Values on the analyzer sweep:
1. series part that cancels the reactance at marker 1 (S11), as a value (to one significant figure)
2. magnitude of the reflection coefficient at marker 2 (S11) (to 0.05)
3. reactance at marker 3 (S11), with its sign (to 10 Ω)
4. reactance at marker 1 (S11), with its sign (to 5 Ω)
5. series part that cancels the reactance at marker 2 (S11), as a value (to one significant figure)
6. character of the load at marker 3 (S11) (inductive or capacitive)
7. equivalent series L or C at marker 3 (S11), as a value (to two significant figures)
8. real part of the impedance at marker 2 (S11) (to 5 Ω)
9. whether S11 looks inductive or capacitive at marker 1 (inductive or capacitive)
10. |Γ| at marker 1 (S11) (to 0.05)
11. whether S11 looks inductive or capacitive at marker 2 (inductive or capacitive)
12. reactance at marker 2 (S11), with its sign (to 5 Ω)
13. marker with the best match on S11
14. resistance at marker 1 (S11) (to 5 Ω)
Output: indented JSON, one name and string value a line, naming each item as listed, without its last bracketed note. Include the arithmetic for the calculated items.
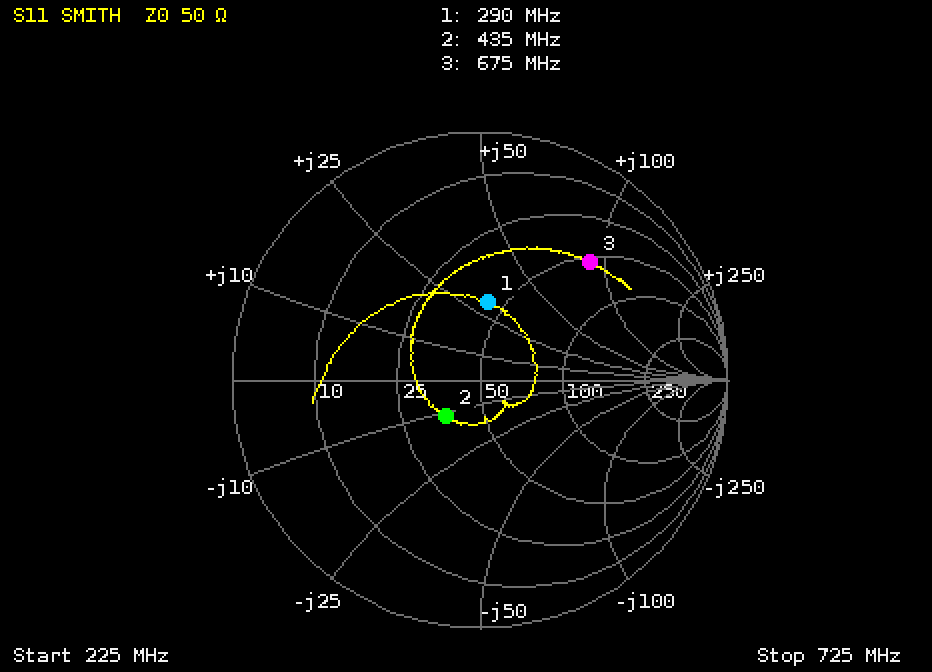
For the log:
{
  "series part that cancels the reactance at marker 1 (S11), as a value": "C = 1/(2π × 290 MHz × 30 Ω) ≈ 18.3 pF, so 20 pF to one significant figure",
  "magnitude of the reflection coefficient at marker 2 (S11)": "0.20",
  "reactance at marker 3 (S11), with its sign": "+90 Ω",
  "reactance at marker 1 (S11), with its sign": "+30 Ω",
  "series part that cancels the reactance at marker 2 (S11), as a value": "L = 10 Ω/(2π × 435 MHz) ≈ 4 nH",
  "character of the load at marker 3 (S11)": "inductive",
  "equivalent series L or C at marker 3 (S11), as a value": "L = 90 Ω/(2π × 675 MHz) ≈ 21 nH",
  "real part of the impedance at marker 2 (S11)": "35 Ω",
  "whether S11 looks inductive or capacitive at marker 1": "inductive",
  "|Γ| at marker 1 (S11)": "0.30",
  "whether S11 looks inductive or capacitive at marker 2": "capacitive",
  "reactance at marker 2 (S11), with its sign": "-10 Ω",
  "marker with the best match on S11": "marker 2",
  "resistance at marker 1 (S11)": "45 Ω"
}
